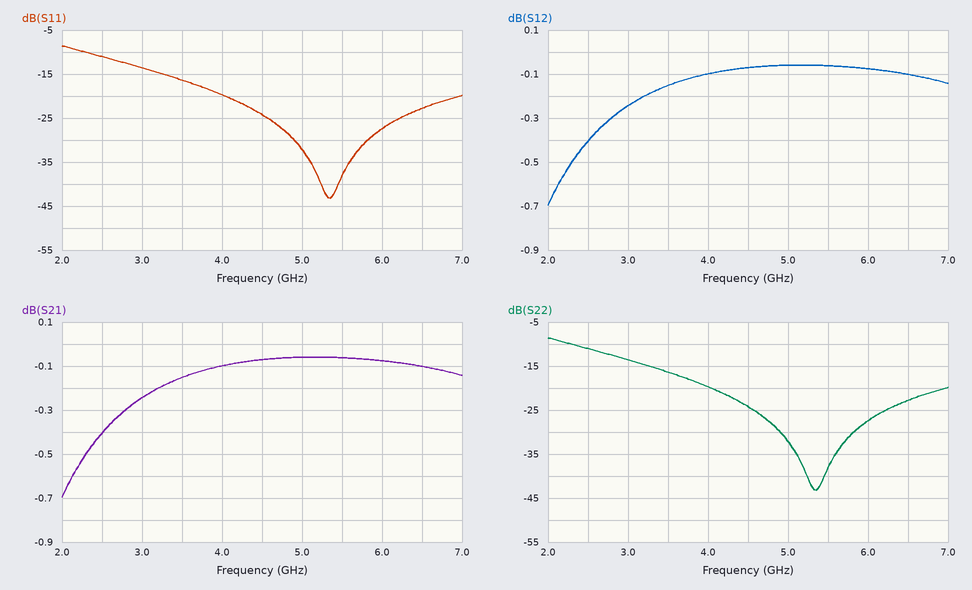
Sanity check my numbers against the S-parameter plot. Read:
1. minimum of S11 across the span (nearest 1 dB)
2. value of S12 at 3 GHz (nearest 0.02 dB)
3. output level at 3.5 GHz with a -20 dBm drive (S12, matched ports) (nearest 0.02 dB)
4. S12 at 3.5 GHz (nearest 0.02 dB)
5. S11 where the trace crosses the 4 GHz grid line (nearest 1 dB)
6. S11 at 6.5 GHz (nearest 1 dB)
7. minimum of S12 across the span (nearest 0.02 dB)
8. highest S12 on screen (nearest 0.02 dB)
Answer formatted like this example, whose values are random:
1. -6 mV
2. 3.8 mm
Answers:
1. -43 dB
2. -0.24 dB
3. -20.16 dBm
4. -0.16 dB
5. -20 dB
6. -23 dB
7. -0.70 dB
8. -0.06 dB
